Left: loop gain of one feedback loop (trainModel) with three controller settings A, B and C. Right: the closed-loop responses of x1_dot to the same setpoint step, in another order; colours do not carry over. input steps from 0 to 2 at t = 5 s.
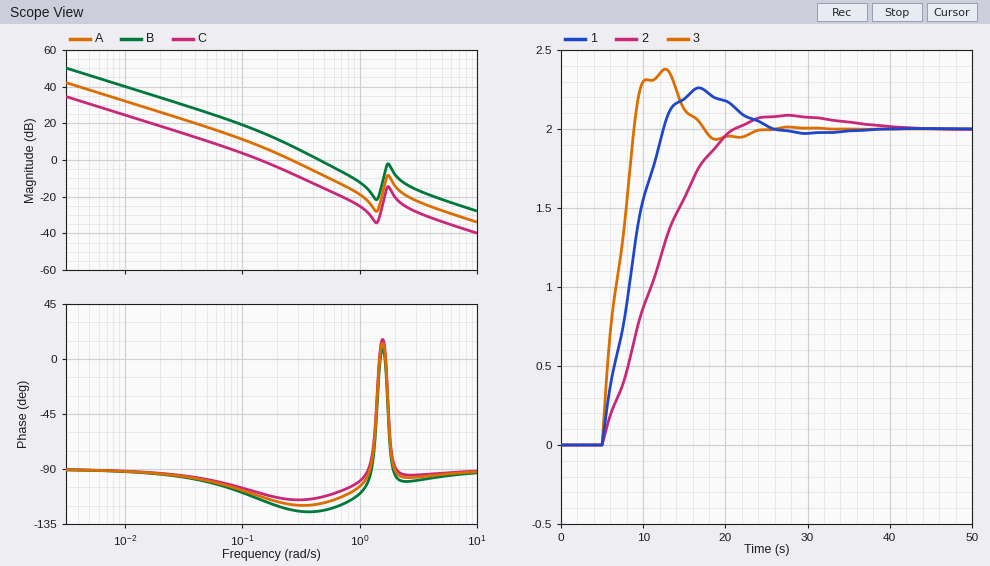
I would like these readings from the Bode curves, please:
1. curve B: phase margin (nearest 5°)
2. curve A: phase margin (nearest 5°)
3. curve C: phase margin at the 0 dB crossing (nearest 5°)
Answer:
55°
60°
70°
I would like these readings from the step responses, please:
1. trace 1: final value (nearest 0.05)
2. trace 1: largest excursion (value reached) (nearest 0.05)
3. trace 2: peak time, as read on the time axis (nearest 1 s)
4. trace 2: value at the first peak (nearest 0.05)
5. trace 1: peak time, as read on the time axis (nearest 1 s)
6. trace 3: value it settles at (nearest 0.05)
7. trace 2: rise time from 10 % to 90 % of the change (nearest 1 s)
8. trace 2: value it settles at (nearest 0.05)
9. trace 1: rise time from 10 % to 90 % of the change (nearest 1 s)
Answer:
2.00
2.25
28 s
2.10
17 s
2.00
11 s
2.00
6 s
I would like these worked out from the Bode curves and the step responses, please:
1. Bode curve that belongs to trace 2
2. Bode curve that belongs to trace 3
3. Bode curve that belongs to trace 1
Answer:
C
B
A
